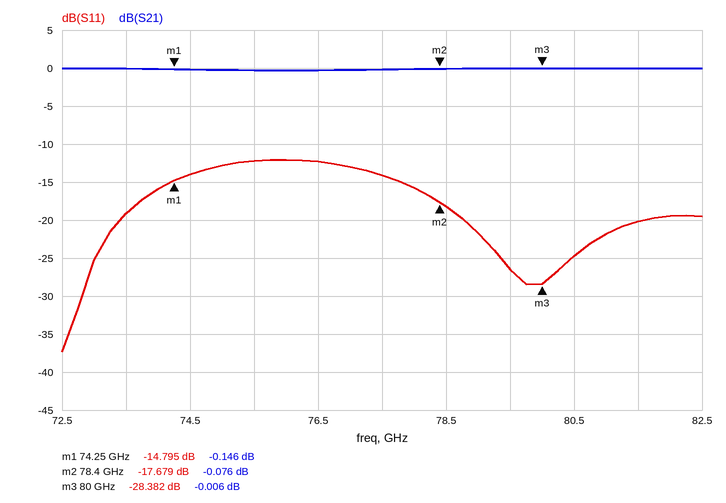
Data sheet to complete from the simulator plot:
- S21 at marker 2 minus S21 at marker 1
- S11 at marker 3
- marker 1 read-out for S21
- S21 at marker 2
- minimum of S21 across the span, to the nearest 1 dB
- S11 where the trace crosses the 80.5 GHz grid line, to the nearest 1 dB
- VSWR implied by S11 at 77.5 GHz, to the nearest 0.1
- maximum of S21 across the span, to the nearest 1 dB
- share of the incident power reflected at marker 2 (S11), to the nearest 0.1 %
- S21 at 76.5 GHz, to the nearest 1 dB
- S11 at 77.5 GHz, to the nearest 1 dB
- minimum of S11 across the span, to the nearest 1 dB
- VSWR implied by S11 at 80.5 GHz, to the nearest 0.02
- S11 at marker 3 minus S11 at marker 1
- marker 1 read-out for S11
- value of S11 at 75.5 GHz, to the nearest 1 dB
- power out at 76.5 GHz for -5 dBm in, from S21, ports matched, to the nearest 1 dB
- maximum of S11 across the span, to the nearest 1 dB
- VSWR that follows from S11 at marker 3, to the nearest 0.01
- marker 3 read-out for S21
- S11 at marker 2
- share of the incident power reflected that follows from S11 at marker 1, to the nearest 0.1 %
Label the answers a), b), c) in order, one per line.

a) 0.070 dB
b) -28.382 dB
c) -0.146 dB
d) -0.076 dB
e) 0 dB
f) -25 dB
g) 1.5
h) 0 dB
i) 1.7 %
j) 0 dB
k) -14 dB
l) -37 dB
m) 1.12
n) -13.587 dB
o) -14.795 dB
p) -12 dB
q) -5 dBm
r) -12 dB
s) 1.08
t) -0.006 dB
u) -17.679 dB
v) 3.3 %
